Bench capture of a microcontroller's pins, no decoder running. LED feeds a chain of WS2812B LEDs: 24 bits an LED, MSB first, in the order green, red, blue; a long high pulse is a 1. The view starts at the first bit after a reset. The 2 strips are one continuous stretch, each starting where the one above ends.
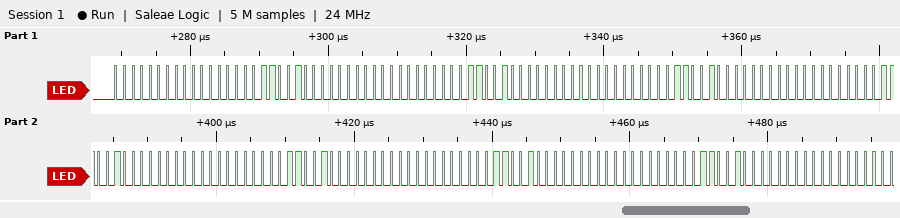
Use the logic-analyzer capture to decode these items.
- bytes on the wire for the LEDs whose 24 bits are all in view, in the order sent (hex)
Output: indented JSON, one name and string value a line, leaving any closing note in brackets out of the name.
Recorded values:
{
  "bytes on the wire for the LEDs whose 24 bits are all in view, in the order sent": "00 00 64 00 00 64 00 00 64 00 00 64 00 00 64 00 00 64 00 00 64"
}
